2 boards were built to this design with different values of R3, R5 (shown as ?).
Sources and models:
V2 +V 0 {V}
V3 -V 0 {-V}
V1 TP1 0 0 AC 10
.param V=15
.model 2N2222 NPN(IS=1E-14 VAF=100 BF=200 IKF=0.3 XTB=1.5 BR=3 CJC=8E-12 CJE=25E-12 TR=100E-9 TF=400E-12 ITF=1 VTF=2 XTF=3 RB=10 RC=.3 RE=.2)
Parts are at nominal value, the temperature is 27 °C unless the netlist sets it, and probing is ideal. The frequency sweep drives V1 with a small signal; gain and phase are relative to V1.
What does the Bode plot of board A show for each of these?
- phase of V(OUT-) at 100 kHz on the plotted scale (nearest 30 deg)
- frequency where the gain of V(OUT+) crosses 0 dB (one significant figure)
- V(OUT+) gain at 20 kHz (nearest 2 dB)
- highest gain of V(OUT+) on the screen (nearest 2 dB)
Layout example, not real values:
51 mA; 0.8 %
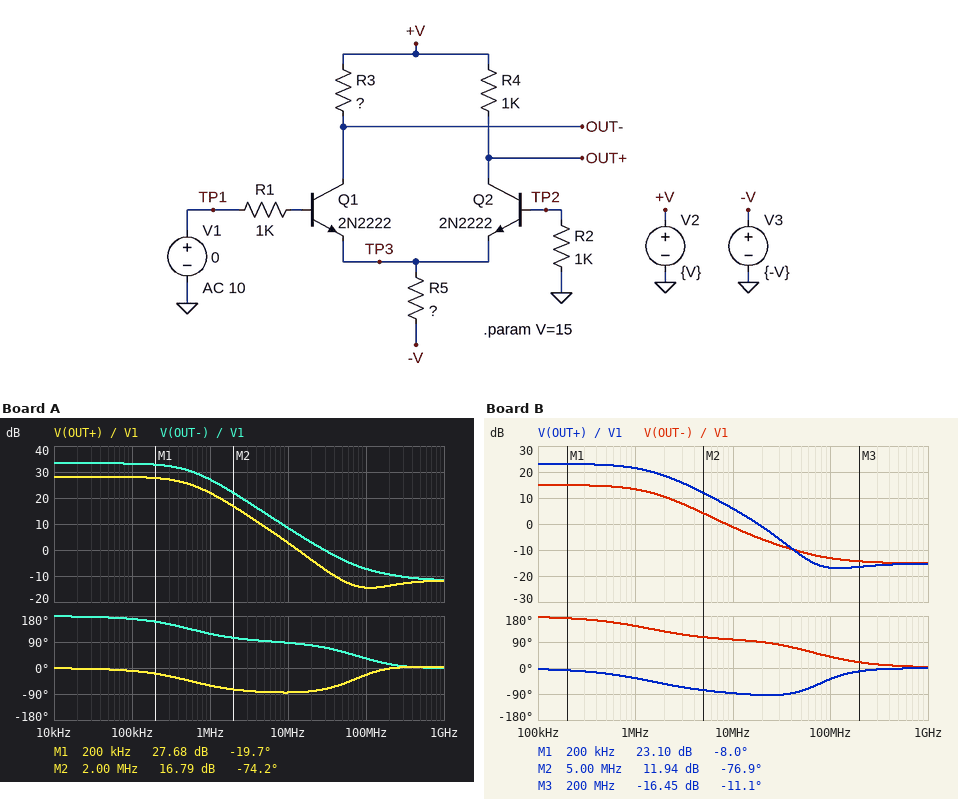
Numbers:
180 deg; 10 MHz; 28 dB; 28 dB
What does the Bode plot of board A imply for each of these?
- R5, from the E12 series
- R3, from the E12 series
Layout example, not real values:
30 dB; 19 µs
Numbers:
3.9 kΩ; 1.8 kΩ
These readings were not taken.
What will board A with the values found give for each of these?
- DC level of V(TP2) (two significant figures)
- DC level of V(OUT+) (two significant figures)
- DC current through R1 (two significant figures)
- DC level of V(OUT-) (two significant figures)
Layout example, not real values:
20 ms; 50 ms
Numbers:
-8.2 mV; 13 V; 8.2 µA; 12 V
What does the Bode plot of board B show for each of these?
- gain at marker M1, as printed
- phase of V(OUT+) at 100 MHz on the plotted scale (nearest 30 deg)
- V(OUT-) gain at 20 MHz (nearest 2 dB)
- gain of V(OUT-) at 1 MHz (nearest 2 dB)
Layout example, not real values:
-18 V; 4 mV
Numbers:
23.10 dB; -30 deg; -6 dB; 14 dB
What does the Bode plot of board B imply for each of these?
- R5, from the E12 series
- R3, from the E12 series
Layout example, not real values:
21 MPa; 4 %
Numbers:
8.2 kΩ; 390 Ω
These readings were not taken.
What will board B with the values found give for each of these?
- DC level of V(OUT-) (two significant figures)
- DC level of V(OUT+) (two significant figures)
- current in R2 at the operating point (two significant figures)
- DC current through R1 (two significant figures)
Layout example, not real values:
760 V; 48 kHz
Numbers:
15 V; 14 V; 3.8 µA; 3.8 µA
